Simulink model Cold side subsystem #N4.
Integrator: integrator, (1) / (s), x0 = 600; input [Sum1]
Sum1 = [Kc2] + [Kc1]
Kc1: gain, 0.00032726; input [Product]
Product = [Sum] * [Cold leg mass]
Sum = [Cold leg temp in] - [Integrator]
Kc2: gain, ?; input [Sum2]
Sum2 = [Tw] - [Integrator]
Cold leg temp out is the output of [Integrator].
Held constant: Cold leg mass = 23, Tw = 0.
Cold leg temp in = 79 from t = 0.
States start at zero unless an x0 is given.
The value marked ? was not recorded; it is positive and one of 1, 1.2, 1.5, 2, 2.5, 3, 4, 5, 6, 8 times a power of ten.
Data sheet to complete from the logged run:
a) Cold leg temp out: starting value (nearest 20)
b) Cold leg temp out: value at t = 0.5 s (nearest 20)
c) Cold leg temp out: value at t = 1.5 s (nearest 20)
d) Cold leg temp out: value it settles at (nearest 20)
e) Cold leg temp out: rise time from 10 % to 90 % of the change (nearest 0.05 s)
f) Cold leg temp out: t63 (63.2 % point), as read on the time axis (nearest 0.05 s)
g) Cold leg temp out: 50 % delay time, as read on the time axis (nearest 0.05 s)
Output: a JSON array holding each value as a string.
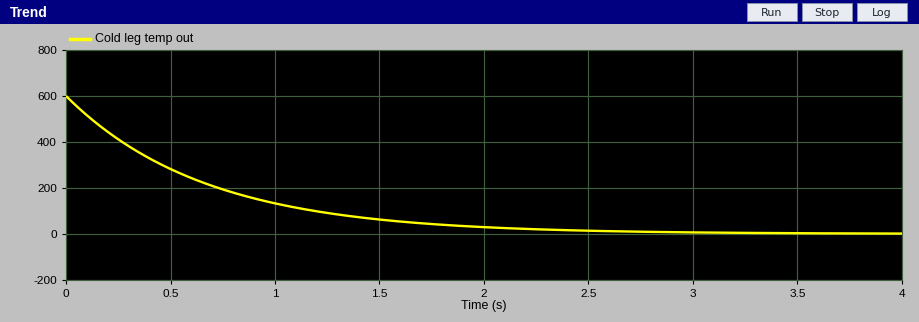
["600", "280", "60", "0", "1.45 s", "0.65 s", "0.45 s"]
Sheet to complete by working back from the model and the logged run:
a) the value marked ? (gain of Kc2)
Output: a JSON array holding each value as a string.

["1.5"]
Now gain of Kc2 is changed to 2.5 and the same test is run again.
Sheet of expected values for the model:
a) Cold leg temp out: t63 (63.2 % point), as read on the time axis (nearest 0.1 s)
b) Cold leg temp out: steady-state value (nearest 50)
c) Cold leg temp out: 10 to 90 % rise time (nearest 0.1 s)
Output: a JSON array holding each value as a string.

["0.4 s", "0", "0.9 s"]
